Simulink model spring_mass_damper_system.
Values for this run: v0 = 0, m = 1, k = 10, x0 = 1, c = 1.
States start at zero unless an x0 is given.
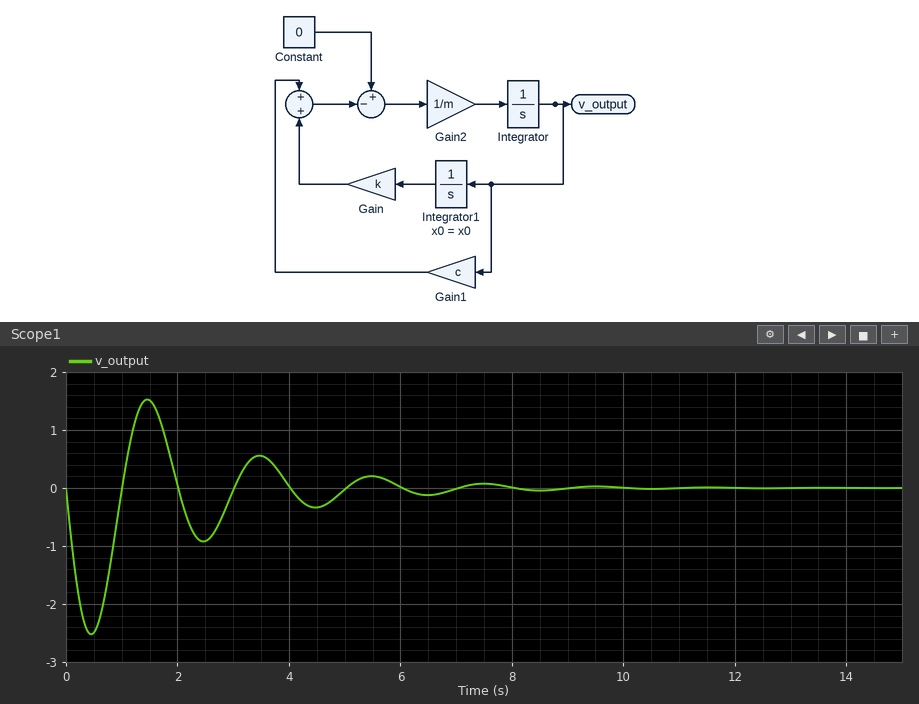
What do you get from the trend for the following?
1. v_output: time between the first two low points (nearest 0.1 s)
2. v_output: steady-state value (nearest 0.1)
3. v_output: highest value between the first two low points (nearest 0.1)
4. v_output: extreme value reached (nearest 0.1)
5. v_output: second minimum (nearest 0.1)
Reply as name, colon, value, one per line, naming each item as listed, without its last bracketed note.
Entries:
v_output: time between the first two low points: 2.0 s
v_output: steady-state value: 0.0
v_output: highest value between the first two low points: 1.5
v_output: extreme value reached: -2.5
v_output: second minimum: -0.9
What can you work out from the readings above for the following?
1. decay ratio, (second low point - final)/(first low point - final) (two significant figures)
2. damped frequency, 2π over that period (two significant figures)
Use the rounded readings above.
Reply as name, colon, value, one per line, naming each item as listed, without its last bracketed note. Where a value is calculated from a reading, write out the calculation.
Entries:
decay ratio, (second low point - final)/(first low point - final): (-0.9 - 0) / (-2.5 - 0) = 0.36
damped frequency, 2π over that period: 2π / 2 = 3.1 rad/s
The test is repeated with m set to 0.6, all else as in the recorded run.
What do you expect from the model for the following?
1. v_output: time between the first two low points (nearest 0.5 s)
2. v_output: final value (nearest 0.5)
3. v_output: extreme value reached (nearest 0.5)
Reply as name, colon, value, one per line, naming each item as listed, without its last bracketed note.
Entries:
v_output: time between the first two low points: 1.5 s
v_output: final value: 0.0
v_output: extreme value reached: -3.0
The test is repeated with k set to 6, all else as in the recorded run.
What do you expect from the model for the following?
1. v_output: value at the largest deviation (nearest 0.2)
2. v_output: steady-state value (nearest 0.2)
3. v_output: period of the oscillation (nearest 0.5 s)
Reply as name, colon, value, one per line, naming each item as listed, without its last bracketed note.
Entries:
v_output: value at the largest deviation: -1.8
v_output: steady-state value: 0.0
v_output: period of the oscillation: 2.5 s
